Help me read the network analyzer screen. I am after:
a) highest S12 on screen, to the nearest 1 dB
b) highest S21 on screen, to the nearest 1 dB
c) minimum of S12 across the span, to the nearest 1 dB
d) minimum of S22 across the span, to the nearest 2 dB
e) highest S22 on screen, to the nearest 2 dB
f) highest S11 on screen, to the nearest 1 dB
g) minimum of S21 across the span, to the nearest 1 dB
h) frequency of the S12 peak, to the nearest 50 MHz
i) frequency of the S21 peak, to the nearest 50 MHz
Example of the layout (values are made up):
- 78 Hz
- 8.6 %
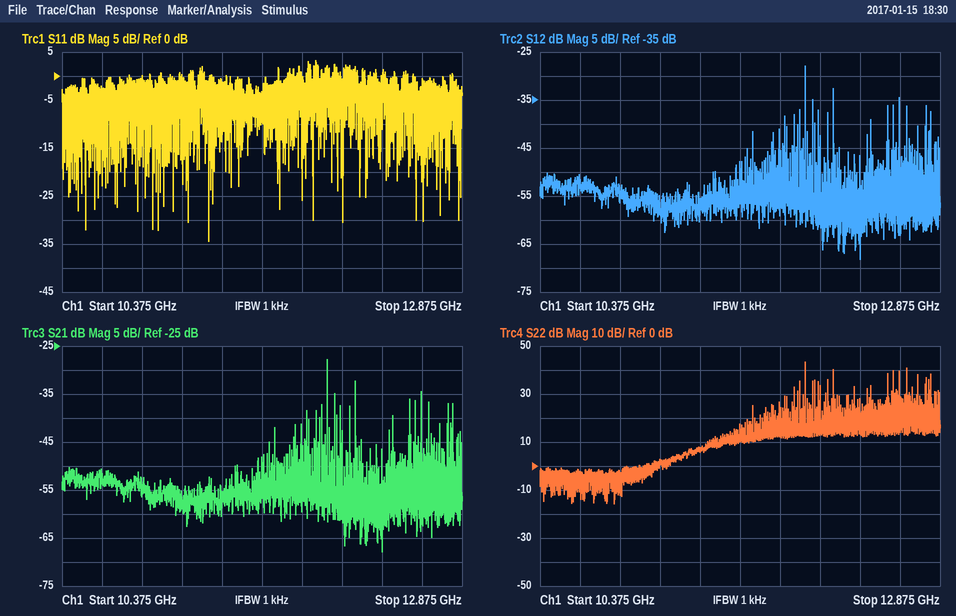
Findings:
- -28 dB
- -28 dB
- -68 dB
- -16 dB
- 44 dB
- 3 dB
- -68 dB
- 12.05 GHz
- 12.05 GHz
